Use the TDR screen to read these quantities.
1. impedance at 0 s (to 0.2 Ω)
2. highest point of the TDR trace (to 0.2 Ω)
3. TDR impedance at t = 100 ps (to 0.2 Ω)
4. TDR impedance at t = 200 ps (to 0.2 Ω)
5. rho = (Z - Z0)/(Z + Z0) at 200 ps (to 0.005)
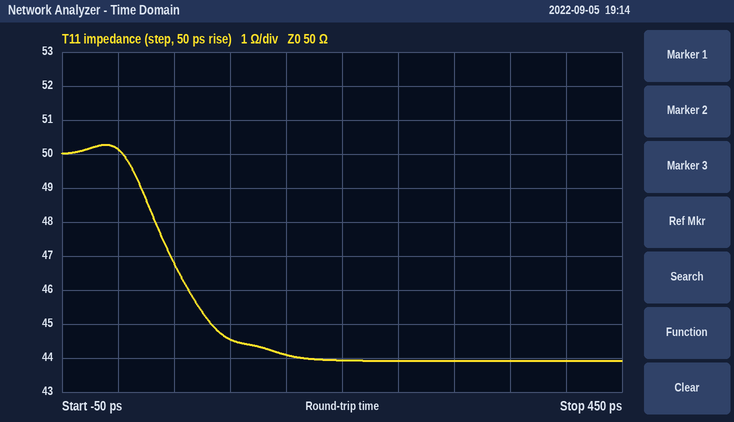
50.2 Ω
50.2 Ω
44.6 Ω
44.0 Ω
-0.065
